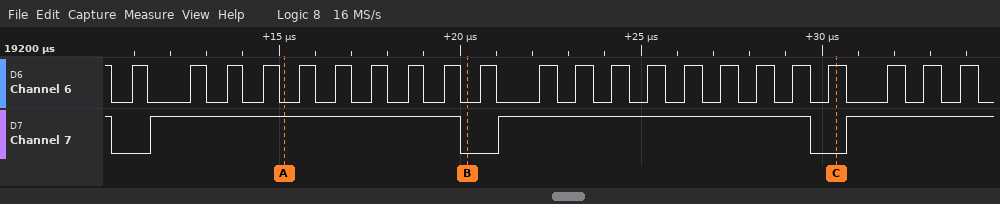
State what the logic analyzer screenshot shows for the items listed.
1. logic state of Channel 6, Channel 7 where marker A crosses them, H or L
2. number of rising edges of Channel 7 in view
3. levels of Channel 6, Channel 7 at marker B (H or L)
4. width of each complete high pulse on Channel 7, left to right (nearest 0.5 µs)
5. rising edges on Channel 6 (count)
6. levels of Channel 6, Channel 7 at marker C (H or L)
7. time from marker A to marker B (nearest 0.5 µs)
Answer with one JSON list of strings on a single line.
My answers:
["Channel 6=L, Channel 7=H", "3", "Channel 6=L, Channel 7=L", "8.5 µs, 8.5 µs", "22", "Channel 6=H, Channel 7=L", "5 µs"]
